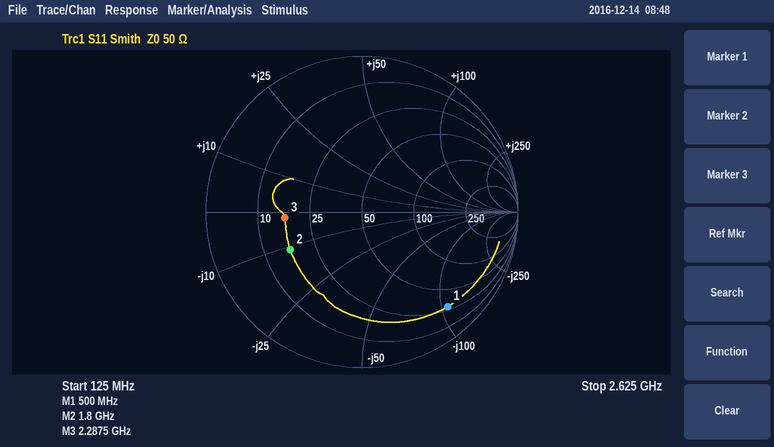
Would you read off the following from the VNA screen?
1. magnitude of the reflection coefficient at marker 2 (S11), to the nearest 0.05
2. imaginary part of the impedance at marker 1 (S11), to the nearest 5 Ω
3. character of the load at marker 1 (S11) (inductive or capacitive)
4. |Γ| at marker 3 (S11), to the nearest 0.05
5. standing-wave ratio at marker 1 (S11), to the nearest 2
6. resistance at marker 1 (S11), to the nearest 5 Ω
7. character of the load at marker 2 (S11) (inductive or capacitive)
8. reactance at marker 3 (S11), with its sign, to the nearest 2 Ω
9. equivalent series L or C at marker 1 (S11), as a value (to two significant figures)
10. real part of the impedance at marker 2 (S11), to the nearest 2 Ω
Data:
0.50
-105 Ω
capacitive
0.50
10
30 Ω
capacitive
-2 Ω
3.0 pF
16 Ω
